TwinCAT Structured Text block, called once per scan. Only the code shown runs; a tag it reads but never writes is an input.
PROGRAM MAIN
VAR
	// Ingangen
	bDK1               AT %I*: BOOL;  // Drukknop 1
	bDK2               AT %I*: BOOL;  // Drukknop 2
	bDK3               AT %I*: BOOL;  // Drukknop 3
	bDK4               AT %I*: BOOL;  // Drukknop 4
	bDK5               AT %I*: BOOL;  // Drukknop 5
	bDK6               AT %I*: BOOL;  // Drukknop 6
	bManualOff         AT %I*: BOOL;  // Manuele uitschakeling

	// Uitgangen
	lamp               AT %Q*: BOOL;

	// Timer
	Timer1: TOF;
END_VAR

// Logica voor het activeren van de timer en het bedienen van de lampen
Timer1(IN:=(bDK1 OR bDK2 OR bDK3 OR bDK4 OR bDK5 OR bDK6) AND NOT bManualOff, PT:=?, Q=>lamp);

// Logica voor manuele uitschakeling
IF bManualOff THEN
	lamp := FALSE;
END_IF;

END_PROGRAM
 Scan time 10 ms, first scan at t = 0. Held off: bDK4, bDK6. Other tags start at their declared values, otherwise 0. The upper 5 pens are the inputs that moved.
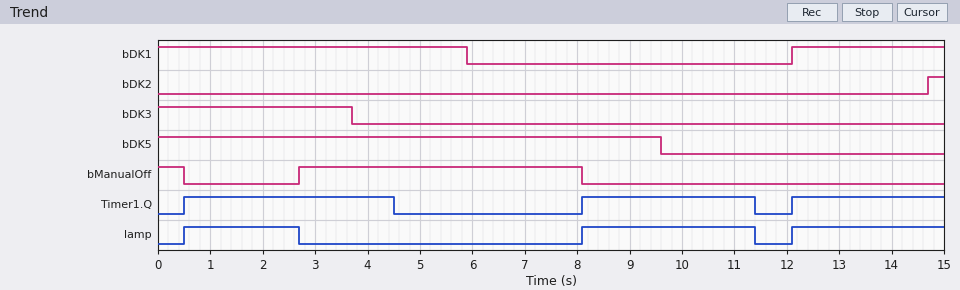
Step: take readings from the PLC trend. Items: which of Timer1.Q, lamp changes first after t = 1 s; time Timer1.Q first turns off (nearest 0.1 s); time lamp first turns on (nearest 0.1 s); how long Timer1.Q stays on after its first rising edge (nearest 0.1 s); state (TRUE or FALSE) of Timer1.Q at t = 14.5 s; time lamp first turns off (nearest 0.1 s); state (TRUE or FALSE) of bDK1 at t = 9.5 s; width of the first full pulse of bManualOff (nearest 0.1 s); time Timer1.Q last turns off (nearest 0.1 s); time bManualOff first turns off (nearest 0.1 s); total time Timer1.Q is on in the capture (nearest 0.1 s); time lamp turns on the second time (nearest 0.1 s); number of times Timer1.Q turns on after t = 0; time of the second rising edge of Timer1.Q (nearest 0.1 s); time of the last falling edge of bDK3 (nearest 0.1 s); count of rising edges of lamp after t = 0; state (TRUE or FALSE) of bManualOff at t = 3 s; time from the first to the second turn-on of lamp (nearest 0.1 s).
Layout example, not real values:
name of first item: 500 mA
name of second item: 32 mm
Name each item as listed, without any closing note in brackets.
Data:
which of Timer1.Q, lamp changes first after t = 1 s: lamp
time Timer1.Q first turns off: 4.5 s
time lamp first turns on: 0.5 s
how long Timer1.Q stays on after its first rising edge: 4.0 s
state (TRUE or FALSE) of Timer1.Q at t = 14.5 s: TRUE
time lamp first turns off: 2.7 s
state (TRUE or FALSE) of bDK1 at t = 9.5 s: FALSE
width of the first full pulse of bManualOff: 5.4 s
time Timer1.Q last turns off: 11.4 s
time bManualOff first turns off: 0.5 s
total time Timer1.Q is on in the capture: 10.2 s
time lamp turns on the second time: 8.1 s
number of times Timer1.Q turns on after t = 0: 3
time of the second rising edge of Timer1.Q: 8.1 s
time of the last falling edge of bDK3: 3.7 s
count of rising edges of lamp after t = 0: 3
state (TRUE or FALSE) of bManualOff at t = 3 s: TRUE
time from the first to the second turn-on of lamp: 7.6 s
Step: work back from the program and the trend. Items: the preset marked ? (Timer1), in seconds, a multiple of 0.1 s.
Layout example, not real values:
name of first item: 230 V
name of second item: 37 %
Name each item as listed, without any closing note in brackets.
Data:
the preset marked ? (Timer1), in seconds, a multiple of 0.1 s: 1.8 s
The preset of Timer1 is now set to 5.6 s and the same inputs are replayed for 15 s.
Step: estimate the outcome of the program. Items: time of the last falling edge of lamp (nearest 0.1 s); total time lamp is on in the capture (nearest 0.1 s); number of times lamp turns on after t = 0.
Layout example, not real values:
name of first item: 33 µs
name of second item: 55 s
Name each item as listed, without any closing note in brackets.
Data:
time of the last falling edge of lamp: 2.7 s
total time lamp is on in the capture: 9.1 s
number of times lamp turns on after t = 0: 2
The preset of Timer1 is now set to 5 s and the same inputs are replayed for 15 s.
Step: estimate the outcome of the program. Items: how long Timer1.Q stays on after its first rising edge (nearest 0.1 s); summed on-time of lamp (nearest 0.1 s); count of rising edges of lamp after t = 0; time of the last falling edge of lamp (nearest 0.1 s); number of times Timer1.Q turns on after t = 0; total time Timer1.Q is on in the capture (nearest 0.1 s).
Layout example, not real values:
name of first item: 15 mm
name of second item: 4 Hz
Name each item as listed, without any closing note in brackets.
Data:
how long Timer1.Q stays on after its first rising edge: 7.2 s
summed on-time of lamp: 9.1 s
count of rising edges of lamp after t = 0: 2
time of the last falling edge of lamp: 2.7 s
number of times Timer1.Q turns on after t = 0: 2
total time Timer1.Q is on in the capture: 14.1 s
